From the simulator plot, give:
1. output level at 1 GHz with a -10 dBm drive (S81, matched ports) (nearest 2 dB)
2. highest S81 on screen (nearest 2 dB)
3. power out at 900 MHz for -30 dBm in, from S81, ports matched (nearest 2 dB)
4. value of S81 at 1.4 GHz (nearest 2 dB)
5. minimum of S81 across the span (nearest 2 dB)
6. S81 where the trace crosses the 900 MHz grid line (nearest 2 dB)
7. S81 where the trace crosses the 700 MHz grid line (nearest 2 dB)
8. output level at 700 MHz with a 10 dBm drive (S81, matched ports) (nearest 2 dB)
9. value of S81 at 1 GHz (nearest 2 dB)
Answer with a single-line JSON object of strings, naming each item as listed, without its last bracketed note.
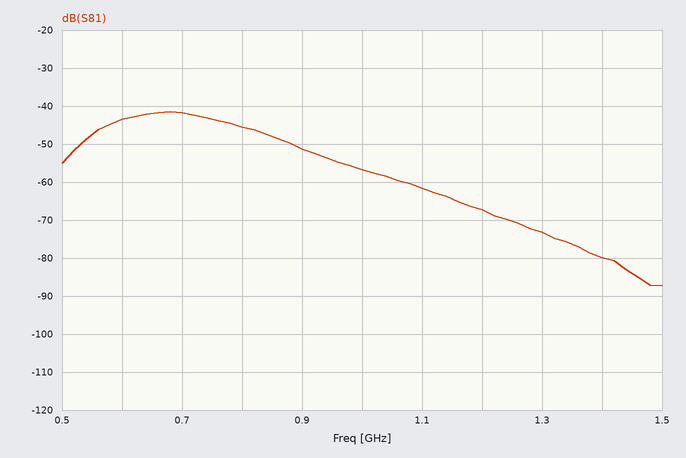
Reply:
{"output level at 1 GHz with a -10 dBm drive (S81, matched ports)": "-66 dBm", "highest S81 on screen": "-42 dB", "power out at 900 MHz for -30 dBm in, from S81, ports matched": "-82 dBm", "value of S81 at 1.4 GHz": "-80 dB", "minimum of S81 across the span": "-88 dB", "S81 where the trace crosses the 900 MHz grid line": "-52 dB", "S81 where the trace crosses the 700 MHz grid line": "-42 dB", "output level at 700 MHz with a 10 dBm drive (S81, matched ports)": "-32 dBm", "value of S81 at 1 GHz": "-56 dB"}
